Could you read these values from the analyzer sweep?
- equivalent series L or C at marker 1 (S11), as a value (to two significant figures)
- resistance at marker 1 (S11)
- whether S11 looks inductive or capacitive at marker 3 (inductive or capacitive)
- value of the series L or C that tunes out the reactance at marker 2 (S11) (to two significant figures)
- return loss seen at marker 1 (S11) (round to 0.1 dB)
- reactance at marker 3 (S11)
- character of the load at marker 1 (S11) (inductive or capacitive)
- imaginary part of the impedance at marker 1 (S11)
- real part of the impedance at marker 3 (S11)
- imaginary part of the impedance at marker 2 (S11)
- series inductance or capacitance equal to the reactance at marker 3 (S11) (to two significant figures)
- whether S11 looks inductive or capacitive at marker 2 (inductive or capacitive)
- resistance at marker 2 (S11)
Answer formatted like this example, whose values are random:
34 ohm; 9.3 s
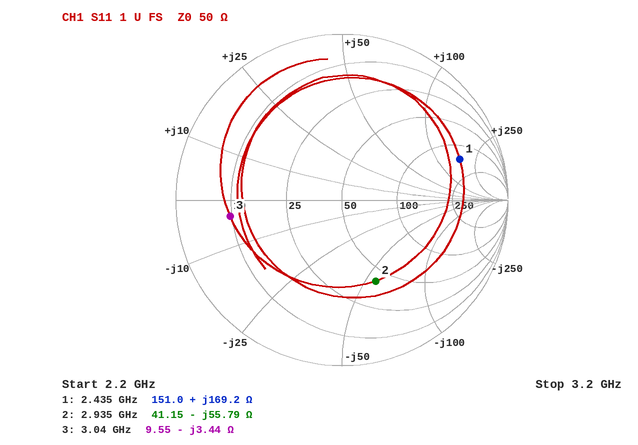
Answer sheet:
11 nH; 151.0 Ω; capacitive; 3.0 nH; 2.5 dB; -3.44 Ω; inductive; +169.2 Ω; 9.55 Ω; -55.79 Ω; 15 pF; capacitive; 41.15 Ω
